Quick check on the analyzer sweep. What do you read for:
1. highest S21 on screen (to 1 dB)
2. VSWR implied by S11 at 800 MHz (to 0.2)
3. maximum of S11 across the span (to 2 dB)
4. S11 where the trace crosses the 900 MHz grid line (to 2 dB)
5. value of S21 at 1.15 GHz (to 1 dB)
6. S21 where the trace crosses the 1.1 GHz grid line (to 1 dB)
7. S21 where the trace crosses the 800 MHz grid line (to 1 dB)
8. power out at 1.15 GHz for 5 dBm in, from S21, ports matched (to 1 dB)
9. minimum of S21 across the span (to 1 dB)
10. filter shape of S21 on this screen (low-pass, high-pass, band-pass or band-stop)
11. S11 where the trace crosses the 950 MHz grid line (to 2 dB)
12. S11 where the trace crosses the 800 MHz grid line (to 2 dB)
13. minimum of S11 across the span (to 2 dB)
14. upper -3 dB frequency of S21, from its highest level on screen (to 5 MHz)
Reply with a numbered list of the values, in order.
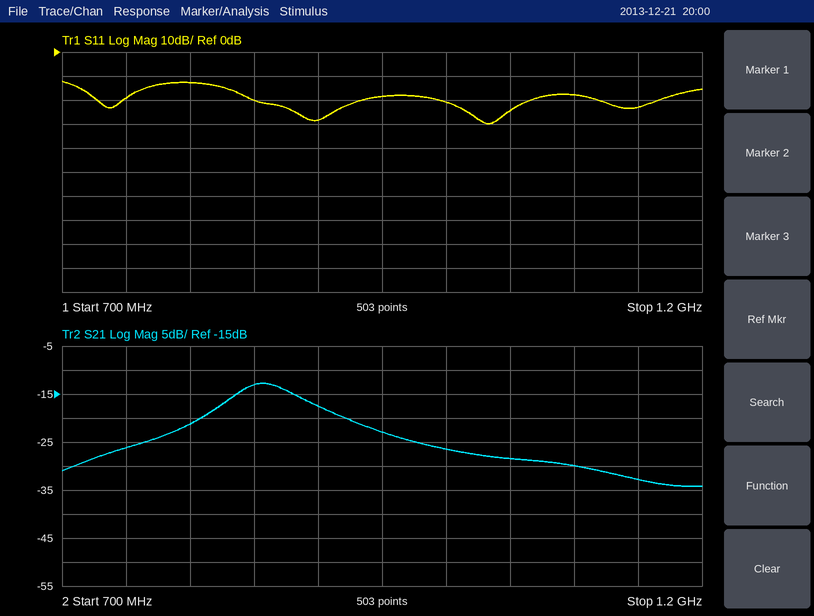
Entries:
1. -13 dB
2. 1.6
3. -12 dB
4. -28 dB
5. -33 dB
6. -30 dB
7. -21 dB
8. -28 dBm
9. -34 dB
10. band-pass
11. -18 dB
12. -12 dB
13. -30 dB
14. 885 MHz
